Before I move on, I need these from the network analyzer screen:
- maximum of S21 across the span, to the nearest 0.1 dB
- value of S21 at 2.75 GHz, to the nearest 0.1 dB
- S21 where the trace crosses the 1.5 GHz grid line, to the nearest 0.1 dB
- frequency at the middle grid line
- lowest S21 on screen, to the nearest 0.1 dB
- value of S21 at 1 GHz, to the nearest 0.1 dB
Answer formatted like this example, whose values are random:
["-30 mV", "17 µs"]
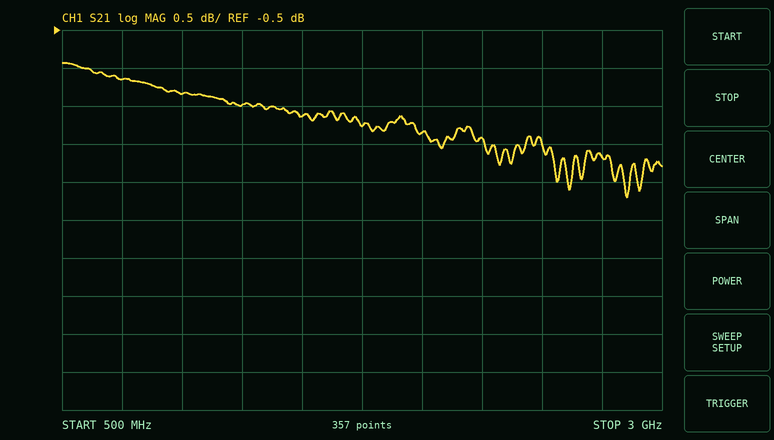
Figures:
["-0.9 dB", "-2.2 dB", "-1.6 dB", "1.75 GHz", "-2.7 dB", "-1.3 dB"]
